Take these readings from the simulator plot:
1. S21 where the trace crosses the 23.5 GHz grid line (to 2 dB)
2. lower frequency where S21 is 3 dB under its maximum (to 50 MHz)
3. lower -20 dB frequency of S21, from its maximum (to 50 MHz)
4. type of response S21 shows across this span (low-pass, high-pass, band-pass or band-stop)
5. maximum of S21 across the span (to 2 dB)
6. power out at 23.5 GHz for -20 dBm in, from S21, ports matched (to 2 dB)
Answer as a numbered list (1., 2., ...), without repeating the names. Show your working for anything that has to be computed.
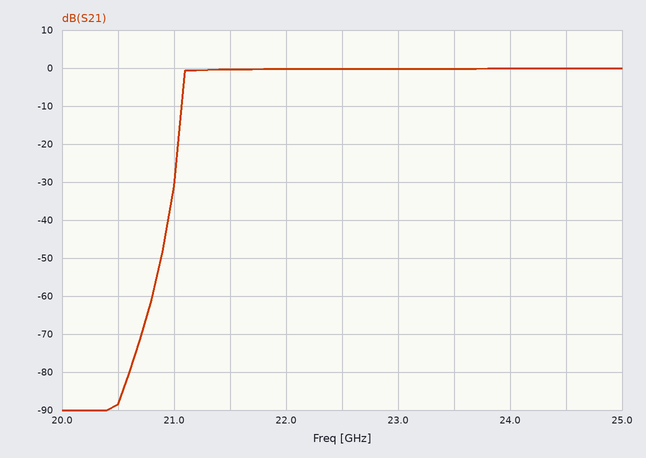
1. 0 dB
2. 21.10 GHz
3. 21.05 GHz
4. high-pass
5. 0 dB
6. -20 dBm + (0 dB) = -20 dBm
